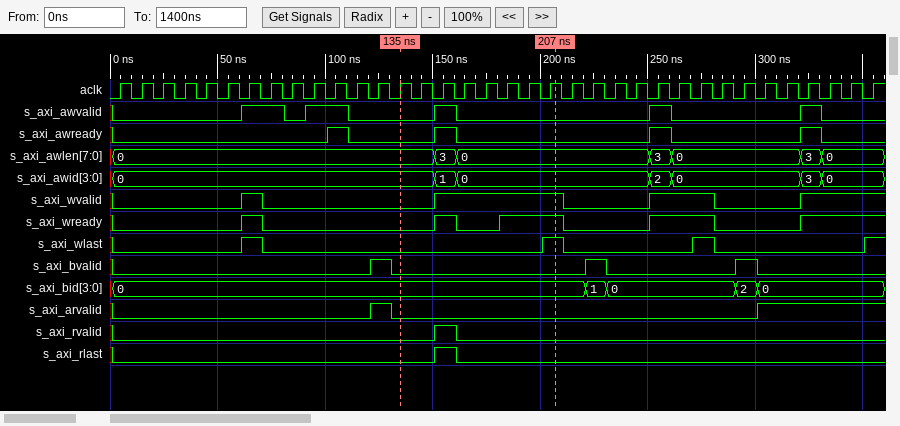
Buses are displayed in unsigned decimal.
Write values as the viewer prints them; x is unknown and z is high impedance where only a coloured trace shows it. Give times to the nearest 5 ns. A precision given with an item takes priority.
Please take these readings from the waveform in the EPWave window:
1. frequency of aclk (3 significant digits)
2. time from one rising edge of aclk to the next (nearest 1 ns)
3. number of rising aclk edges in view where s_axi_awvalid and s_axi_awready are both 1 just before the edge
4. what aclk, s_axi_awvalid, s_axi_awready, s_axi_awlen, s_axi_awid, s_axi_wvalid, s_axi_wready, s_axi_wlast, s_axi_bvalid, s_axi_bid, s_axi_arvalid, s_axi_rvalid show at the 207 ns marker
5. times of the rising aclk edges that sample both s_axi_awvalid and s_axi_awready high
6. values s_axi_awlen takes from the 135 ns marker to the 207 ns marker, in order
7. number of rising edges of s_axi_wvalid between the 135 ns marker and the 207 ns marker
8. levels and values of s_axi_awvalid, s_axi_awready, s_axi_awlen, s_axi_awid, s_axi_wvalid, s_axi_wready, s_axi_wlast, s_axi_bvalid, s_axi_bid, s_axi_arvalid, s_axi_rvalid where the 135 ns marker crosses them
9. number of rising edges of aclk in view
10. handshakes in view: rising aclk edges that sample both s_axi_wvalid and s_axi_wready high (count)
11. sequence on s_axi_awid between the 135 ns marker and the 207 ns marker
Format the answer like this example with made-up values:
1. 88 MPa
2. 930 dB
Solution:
1. 100 MHz
2. 10 ns
3. 4
4. aclk=1, s_axi_awvalid=0, s_axi_awready=0, s_axi_awlen=0, s_axi_awid=0, s_axi_wvalid=1, s_axi_wready=1, s_axi_wlast=1, s_axi_bvalid=0, s_axi_bid=0, s_axi_arvalid=0, s_axi_rvalid=0
5. 105 ns, 155 ns, 255 ns, 325 ns
6. 0, 3, 0
7. 1
8. s_axi_awvalid=0, s_axi_awready=0, s_axi_awlen=0, s_axi_awid=0, s_axi_wvalid=0, s_axi_wready=0, s_axi_wlast=0, s_axi_bvalid=0, s_axi_bid=0, s_axi_arvalid=0, s_axi_rvalid=0
9. 36
10. 12
11. 0, 1, 0
